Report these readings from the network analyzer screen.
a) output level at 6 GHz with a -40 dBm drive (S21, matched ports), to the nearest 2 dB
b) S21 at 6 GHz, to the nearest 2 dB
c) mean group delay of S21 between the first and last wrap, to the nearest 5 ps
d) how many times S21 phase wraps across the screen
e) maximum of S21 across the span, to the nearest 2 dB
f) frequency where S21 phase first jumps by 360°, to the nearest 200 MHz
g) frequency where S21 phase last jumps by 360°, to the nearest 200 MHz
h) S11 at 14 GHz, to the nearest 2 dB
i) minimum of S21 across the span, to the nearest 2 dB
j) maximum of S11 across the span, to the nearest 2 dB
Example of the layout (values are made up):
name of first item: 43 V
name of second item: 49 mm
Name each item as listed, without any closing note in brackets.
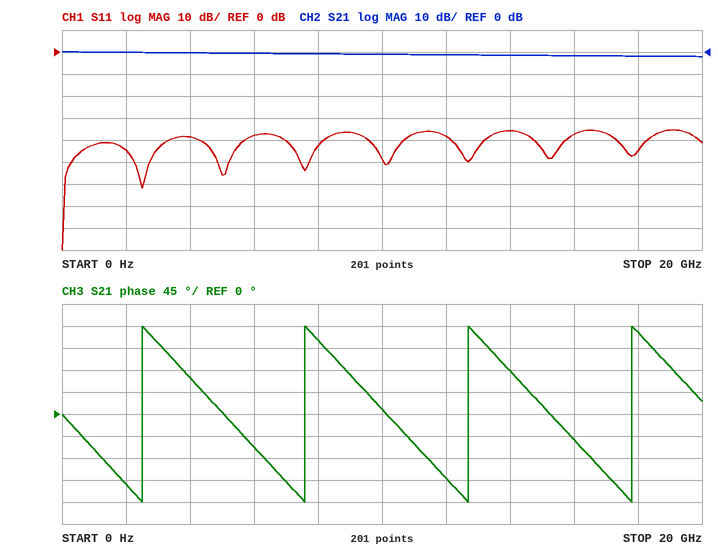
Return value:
output level at 6 GHz with a -40 dBm drive (S21, matched ports), to the nearest 2 dB: -40 dBm
S21 at 6 GHz, to the nearest 2 dB: 0 dB
mean group delay of S21 between the first and last wrap, to the nearest 5 ps: 195 ps
how many times S21 phase wraps across the screen: 4
maximum of S21 across the span, to the nearest 2 dB: 0 dB
frequency where S21 phase first jumps by 360°, to the nearest 200 MHz: 2.6 GHz
frequency where S21 phase last jumps by 360°, to the nearest 200 MHz: 17.8 GHz
S11 at 14 GHz, to the nearest 2 dB: -36 dB
minimum of S21 across the span, to the nearest 2 dB: -2 dB
maximum of S11 across the span, to the nearest 2 dB: -36 dB
